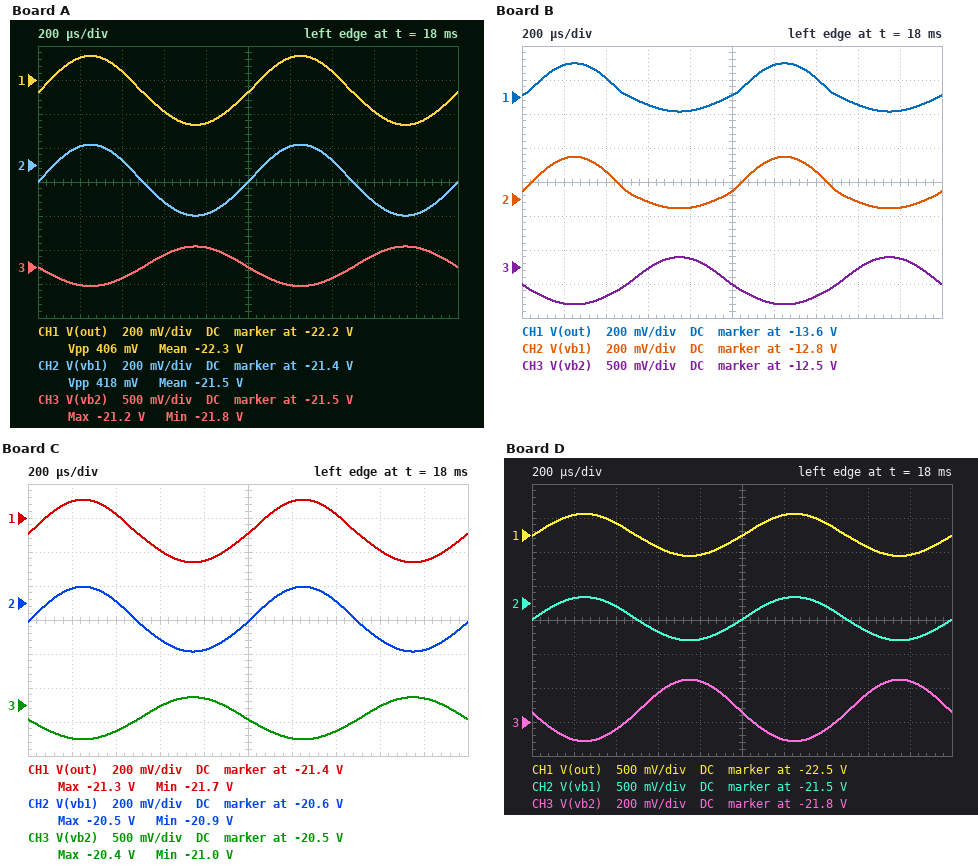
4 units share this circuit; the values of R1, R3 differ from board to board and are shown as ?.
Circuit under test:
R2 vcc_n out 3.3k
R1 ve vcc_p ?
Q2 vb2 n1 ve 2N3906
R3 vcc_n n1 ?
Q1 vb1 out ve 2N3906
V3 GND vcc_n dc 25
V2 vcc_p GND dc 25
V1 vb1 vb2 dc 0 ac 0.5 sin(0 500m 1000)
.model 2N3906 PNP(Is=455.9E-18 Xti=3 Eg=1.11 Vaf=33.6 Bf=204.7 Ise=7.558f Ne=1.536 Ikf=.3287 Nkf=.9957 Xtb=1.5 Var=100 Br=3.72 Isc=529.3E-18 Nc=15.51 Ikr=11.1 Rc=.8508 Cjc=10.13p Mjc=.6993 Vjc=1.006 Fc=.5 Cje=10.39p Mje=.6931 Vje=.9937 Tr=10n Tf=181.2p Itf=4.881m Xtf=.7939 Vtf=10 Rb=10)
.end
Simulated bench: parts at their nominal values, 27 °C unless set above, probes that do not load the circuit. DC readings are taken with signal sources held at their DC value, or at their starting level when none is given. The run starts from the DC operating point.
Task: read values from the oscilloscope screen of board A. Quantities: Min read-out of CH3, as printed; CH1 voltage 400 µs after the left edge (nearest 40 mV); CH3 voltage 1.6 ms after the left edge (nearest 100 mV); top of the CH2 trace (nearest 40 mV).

-21.8 V
-22.16 V
-21.3 V
-21.28 V
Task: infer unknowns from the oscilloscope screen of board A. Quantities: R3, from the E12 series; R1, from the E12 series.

4.7 kΩ
33 kΩ
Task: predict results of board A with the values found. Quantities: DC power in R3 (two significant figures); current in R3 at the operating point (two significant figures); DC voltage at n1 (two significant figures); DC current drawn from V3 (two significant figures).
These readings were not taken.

1.6 mW
580 µA
-22 V
1.4 mA
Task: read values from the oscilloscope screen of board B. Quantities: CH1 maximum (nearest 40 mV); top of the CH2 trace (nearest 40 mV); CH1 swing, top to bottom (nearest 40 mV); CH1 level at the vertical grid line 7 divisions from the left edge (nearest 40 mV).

-13.40 V
-12.56 V
280 mV
-13.48 V
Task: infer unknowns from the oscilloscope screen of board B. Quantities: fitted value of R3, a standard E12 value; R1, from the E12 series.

10 kΩ
8.2 kΩ
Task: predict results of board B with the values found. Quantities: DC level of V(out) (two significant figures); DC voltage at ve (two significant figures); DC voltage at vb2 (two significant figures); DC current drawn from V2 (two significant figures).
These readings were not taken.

-14 V
-13 V
-13 V
4.6 mA
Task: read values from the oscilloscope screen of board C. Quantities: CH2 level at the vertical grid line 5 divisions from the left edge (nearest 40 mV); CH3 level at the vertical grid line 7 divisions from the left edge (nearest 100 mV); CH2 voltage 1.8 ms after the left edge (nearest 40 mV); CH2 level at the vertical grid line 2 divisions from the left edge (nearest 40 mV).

-20.72 V
-20.9 V
-20.88 V
-20.60 V
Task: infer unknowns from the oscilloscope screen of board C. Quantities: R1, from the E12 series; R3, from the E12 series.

27 kΩ
5.6 kΩ
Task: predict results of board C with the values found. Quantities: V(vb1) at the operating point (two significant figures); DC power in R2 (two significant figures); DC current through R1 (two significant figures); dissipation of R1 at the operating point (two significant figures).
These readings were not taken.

-21 V
3.7 mW
1.7 mA
77 mW
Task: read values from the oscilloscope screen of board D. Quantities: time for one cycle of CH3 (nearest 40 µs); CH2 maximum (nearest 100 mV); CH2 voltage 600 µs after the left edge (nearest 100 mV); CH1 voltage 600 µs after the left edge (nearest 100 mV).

1.00 ms
-21.4 V
-21.9 V
-22.7 V
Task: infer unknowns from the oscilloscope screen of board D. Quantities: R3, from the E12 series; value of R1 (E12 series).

1.8 kΩ
22 kΩ
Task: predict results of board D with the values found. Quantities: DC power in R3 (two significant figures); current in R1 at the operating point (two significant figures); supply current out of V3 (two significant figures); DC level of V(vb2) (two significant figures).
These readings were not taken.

3.4 mW
2.1 mA
2.1 mA
-22 V
